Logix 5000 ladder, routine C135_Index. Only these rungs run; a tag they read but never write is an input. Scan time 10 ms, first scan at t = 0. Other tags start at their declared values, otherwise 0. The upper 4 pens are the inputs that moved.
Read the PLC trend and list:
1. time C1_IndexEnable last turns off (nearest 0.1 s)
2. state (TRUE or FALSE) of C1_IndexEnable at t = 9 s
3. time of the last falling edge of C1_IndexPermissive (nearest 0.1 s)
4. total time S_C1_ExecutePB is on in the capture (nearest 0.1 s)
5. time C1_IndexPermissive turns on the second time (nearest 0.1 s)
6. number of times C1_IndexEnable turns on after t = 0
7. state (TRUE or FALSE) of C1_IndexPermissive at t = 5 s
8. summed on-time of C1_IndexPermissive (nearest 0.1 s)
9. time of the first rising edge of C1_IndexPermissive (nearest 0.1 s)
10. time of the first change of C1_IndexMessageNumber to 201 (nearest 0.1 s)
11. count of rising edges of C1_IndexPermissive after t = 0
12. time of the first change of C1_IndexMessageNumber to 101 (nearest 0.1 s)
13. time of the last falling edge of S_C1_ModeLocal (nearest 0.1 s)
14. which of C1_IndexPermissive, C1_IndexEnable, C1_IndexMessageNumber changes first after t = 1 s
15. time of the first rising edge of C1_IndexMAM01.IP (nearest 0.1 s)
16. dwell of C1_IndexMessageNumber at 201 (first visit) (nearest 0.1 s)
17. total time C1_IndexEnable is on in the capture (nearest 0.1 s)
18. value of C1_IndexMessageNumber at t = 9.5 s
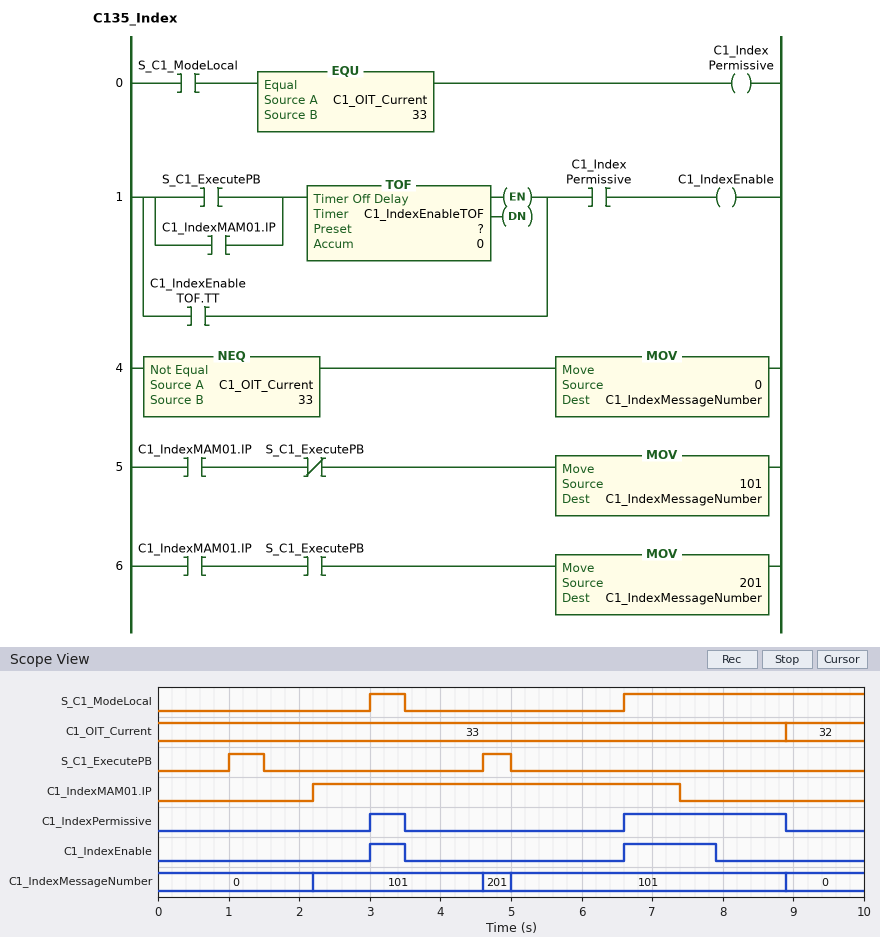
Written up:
7.9 s
FALSE
8.9 s
0.9 s
6.6 s
2
FALSE
2.8 s
3.0 s
4.6 s
2
2.2 s
3.5 s
C1_IndexMessageNumber
2.2 s
0.4 s
1.8 s
0
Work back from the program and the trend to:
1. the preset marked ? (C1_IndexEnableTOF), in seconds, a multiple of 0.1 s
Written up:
0.5 s
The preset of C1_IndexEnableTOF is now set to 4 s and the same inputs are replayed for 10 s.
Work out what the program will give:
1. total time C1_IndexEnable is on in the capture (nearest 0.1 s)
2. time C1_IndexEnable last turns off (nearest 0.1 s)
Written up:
2.8 s
8.9 s
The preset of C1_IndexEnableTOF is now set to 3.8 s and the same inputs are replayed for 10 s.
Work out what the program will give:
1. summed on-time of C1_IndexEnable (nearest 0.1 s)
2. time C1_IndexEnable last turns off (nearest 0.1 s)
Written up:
2.8 s
8.9 s
